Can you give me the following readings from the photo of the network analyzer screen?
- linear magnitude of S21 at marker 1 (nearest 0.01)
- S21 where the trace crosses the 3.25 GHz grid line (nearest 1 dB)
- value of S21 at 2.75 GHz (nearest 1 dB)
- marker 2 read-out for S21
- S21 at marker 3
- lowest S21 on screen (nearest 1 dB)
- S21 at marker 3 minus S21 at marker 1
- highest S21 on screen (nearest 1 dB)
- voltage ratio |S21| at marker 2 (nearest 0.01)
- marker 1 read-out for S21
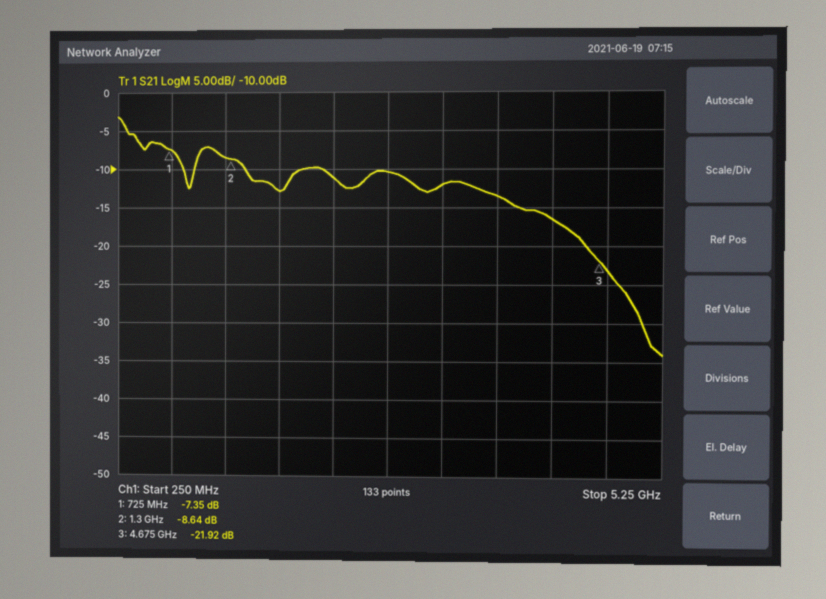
0.43
-12 dB
-10 dB
-8.64 dB
-21.92 dB
-34 dB
-14.57 dB
-3 dB
0.37
-7.35 dB
